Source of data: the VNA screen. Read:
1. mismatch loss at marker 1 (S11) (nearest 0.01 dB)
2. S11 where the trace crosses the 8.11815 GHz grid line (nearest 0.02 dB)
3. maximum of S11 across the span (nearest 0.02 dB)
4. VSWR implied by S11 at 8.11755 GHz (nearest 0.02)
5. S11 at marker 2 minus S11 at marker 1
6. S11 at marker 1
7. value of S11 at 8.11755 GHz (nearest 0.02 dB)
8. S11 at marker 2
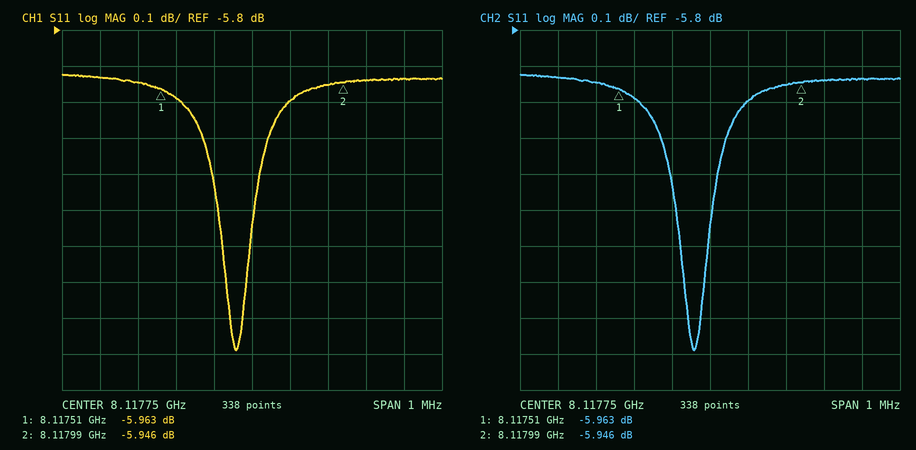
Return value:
1.27 dB
-5.94 dB
-5.92 dB
3.02
0.017 dB
-5.963 dB
-5.98 dB
-5.946 dB
